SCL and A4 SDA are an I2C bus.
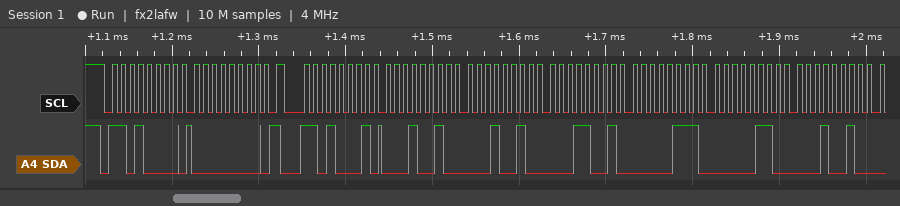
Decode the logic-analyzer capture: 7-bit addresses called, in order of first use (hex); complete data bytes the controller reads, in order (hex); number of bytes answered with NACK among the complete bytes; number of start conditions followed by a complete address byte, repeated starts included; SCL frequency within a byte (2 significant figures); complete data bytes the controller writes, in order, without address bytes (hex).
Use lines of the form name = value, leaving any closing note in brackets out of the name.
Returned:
7-bit addresses called, in order of first use = 0x68
complete data bytes the controller reads, in order = 12 12 19 07 06 12
number of bytes answered with NACK among the complete bytes = 0
number of start conditions followed by a complete address byte, repeated starts included = 2
SCL frequency within a byte = 100 kHz
complete data bytes the controller writes, in order, without address bytes = 00
